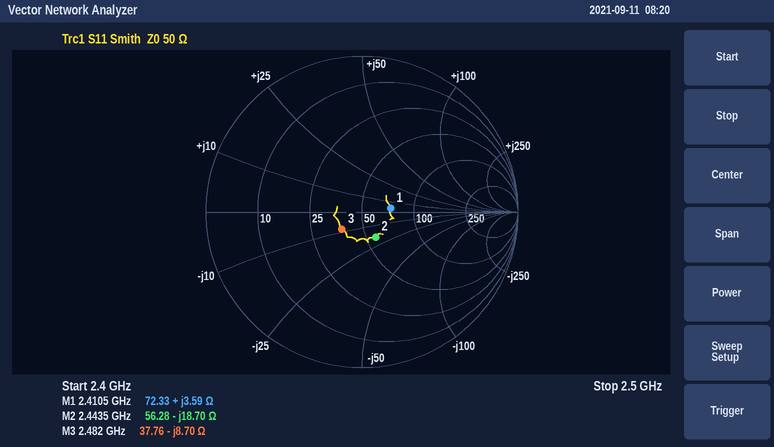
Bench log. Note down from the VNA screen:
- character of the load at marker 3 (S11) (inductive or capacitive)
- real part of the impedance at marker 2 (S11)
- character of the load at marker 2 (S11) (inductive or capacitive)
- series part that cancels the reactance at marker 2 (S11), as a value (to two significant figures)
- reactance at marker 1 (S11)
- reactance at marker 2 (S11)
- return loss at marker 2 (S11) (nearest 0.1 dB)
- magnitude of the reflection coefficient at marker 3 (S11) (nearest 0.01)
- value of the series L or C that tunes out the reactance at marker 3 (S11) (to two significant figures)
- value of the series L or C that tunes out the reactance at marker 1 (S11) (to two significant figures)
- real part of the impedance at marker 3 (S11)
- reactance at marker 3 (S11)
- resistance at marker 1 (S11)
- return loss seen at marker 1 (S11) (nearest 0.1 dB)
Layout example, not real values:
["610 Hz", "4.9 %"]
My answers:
["capacitive", "56.28 Ω", "capacitive", "1.2 nH", "+3.59 Ω", "-18.70 Ω", "14.8 dB", "0.17", "560 pH", "18 pF", "37.76 Ω", "-8.70 Ω", "72.33 Ω", "14.7 dB"]
